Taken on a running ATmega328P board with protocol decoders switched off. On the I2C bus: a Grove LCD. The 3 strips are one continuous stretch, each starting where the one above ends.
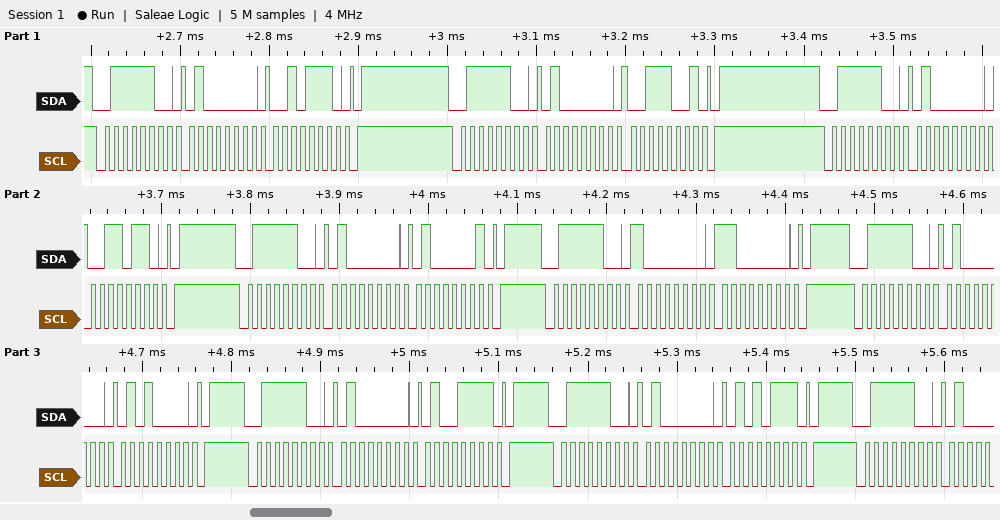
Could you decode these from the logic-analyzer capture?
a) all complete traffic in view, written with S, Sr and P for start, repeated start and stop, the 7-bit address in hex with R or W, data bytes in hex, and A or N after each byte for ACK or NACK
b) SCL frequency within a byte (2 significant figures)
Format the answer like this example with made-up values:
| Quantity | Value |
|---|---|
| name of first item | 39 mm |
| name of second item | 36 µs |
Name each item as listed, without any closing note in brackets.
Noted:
| Quantity | Value |
|---|---|
| all complete traffic in view, written with S, Sr and P for start, repeated start and stop, the 7-bit address in hex with R or W, data bytes in hex, and A or N after each byte for ACK or NACK | S 3EW A 40 A 2E A P S 3EW A 40 A 39 A P S 3EW A 40 A 36 A P S 3EW A 40 A 41 A P S 3EW A 80 A C0 A P S 3EW A 40 A 50 A P S 3EW A 40 A 4F A P S 3EW A 40 A 57 A P S 3EW A |
| SCL frequency within a byte | 100 kHz |
